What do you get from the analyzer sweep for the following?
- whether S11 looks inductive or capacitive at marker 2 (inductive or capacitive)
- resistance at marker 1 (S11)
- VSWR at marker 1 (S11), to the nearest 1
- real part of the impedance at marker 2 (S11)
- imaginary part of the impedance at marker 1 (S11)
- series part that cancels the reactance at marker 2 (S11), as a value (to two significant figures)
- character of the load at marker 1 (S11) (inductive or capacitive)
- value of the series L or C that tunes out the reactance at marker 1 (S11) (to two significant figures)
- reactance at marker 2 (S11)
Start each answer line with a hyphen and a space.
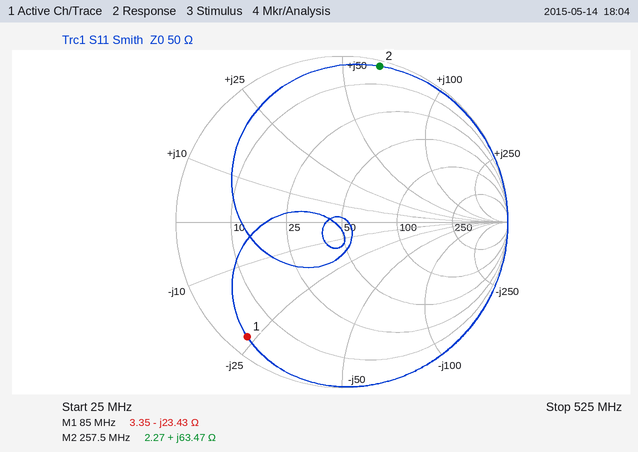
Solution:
- inductive
- 3.35 Ω
- 18
- 2.27 Ω
- -23.43 Ω
- 9.7 pF
- capacitive
- 44 nH
- +63.47 Ω
